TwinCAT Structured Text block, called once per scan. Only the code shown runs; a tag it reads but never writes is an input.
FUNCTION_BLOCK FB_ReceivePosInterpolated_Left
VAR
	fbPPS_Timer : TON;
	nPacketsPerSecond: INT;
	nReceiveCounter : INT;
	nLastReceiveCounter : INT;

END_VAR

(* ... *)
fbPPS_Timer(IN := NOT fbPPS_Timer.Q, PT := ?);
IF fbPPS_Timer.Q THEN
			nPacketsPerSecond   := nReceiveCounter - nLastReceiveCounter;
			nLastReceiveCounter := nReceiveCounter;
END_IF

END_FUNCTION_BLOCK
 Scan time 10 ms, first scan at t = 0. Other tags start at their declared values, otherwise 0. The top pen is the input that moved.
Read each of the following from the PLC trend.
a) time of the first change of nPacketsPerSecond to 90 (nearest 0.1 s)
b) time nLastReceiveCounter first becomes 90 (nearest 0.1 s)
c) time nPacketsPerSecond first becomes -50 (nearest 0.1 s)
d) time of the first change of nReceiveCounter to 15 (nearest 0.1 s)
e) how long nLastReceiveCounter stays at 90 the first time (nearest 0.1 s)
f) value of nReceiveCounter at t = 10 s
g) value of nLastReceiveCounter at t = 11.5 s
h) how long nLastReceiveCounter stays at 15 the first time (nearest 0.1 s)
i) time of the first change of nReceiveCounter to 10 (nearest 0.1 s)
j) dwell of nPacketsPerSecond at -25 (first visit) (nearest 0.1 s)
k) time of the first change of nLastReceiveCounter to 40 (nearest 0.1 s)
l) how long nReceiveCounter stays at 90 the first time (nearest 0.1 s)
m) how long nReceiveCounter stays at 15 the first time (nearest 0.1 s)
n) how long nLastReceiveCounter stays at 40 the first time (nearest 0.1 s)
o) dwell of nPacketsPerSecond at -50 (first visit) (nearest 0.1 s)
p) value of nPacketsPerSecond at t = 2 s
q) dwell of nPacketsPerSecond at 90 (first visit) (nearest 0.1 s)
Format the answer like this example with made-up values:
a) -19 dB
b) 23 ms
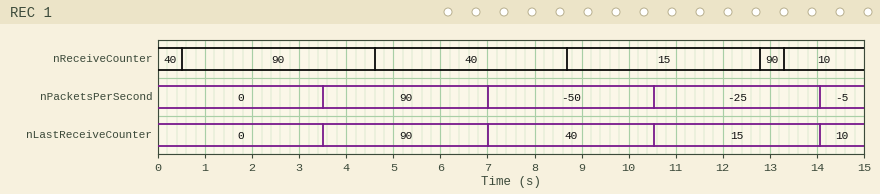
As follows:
a) 3.5 s
b) 3.5 s
c) 7.0 s
d) 8.7 s
e) 3.5 s
f) 15
g) 15
h) 3.5 s
i) 13.3 s
j) 3.5 s
k) 7.0 s
l) 4.1 s
m) 4.1 s
n) 3.5 s
o) 3.5 s
p) 0
q) 3.5 s
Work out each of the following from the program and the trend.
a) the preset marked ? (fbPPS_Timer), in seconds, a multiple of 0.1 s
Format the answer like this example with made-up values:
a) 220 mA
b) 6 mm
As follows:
a) 3.5 s
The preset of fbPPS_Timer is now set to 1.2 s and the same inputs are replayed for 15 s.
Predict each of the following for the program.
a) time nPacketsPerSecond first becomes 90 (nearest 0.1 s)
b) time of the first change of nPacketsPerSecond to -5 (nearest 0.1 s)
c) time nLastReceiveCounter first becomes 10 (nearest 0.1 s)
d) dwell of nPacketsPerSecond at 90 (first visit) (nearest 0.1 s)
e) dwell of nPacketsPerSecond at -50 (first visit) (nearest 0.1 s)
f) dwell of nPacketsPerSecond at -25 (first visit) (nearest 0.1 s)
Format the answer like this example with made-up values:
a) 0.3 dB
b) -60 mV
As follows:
a) 1.2 s
b) 13.4 s
c) 13.4 s
d) 1.2 s
e) 1.2 s
f) 1.2 s
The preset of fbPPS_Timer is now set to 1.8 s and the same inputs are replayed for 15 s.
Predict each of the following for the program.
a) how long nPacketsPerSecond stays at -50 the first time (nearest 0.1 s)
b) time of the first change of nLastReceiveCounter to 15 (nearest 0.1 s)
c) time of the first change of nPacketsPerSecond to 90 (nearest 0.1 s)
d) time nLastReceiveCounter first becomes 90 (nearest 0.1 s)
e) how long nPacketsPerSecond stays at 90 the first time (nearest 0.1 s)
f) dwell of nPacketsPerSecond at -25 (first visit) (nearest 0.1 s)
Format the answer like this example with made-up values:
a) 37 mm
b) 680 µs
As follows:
a) 1.8 s
b) 9.1 s
c) 1.8 s
d) 1.8 s
e) 1.8 s
f) 1.8 s
